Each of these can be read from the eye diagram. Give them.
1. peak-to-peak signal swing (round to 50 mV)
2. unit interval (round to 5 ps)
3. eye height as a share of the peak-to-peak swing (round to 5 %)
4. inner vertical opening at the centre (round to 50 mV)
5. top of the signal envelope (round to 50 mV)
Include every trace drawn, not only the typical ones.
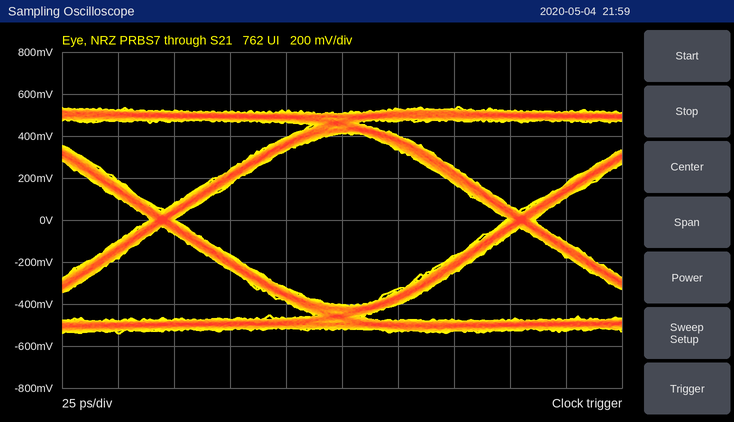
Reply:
1.10 V
160 ps
75 %
800 mV
550 mV
